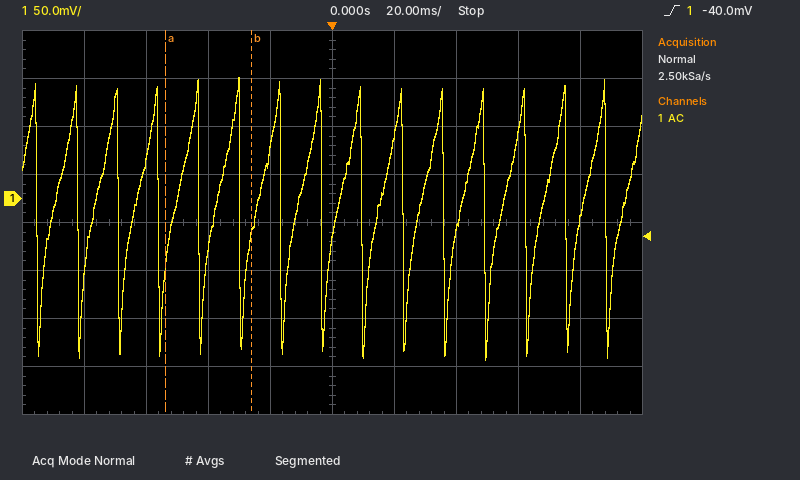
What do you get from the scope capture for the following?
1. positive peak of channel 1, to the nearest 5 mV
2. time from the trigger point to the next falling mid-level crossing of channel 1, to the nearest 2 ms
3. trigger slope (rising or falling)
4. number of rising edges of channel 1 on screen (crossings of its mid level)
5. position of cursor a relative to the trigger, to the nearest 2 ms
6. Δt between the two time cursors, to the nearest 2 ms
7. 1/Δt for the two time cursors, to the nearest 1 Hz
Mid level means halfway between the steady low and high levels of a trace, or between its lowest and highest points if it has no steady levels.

125 mV
10 ms
rising
15
-54 ms
28 ms
36 Hz
